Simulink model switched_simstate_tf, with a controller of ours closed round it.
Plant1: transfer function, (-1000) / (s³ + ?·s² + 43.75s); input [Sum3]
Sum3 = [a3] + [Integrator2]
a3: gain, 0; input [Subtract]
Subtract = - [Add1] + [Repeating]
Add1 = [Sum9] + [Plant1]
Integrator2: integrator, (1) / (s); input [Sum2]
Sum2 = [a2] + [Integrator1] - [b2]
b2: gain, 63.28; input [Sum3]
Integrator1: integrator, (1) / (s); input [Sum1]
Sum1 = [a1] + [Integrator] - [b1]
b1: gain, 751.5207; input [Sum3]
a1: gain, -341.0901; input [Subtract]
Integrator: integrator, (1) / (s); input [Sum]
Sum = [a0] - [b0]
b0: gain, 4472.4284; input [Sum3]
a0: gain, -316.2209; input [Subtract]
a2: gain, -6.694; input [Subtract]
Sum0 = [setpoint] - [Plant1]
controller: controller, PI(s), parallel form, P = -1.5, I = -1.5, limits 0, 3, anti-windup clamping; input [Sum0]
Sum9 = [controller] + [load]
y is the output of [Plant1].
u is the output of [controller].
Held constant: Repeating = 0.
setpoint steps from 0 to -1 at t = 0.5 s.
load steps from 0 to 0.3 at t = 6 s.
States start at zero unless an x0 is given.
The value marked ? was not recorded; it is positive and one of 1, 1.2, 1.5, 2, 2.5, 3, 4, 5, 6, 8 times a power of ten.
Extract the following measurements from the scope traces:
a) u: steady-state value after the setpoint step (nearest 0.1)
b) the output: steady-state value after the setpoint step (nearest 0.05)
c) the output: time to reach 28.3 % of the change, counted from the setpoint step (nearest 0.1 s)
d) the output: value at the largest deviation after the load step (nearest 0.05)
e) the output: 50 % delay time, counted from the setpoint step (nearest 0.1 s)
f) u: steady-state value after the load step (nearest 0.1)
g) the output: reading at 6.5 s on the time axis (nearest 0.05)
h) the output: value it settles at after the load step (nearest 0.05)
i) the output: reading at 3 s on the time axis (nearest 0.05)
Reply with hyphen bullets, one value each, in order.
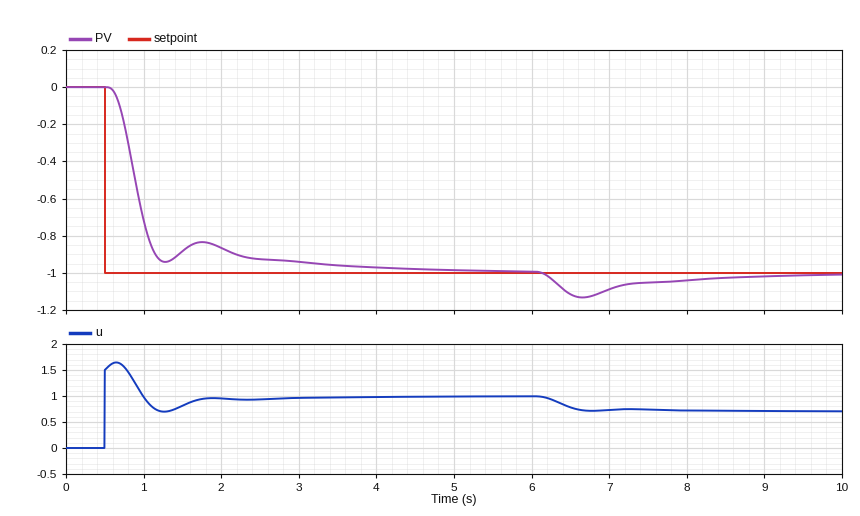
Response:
- 1.0
- -1.00
- 0.3 s
- -1.15
- 0.4 s
- 0.7
- -1.10
- -1.00
- -0.95
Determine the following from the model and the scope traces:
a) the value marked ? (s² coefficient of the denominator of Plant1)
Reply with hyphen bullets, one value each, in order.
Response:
- 50
